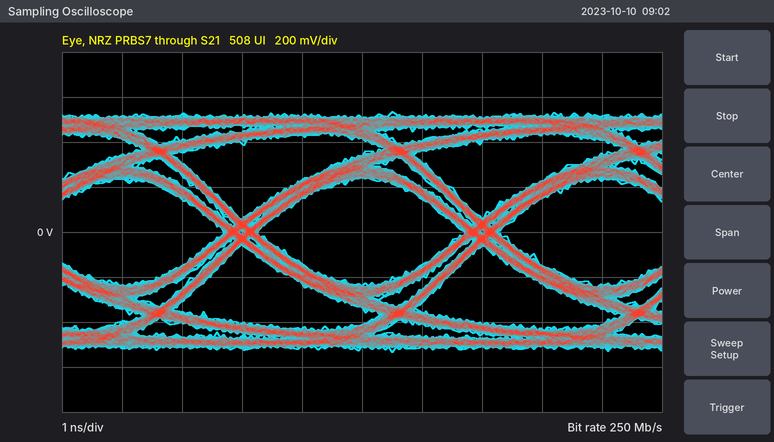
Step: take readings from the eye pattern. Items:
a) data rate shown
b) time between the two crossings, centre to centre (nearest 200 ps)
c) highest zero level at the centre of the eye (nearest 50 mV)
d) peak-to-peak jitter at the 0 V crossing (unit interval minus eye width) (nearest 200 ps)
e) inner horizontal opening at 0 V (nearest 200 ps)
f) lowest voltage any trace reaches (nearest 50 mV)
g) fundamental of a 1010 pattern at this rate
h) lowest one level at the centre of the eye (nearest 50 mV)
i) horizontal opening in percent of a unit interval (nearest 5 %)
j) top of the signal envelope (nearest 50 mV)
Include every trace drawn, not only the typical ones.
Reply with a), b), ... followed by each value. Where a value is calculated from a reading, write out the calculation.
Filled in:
a) 250 Mb/s
b) 4.0 ns
c) -250 mV
d) 600 ps
e) 3.4 ns
f) -550 mV
g) 125 MHz
h) 250 mV
i) 3.4 ns / 4.0 ns ≈ 85 %
j) 550 mV
